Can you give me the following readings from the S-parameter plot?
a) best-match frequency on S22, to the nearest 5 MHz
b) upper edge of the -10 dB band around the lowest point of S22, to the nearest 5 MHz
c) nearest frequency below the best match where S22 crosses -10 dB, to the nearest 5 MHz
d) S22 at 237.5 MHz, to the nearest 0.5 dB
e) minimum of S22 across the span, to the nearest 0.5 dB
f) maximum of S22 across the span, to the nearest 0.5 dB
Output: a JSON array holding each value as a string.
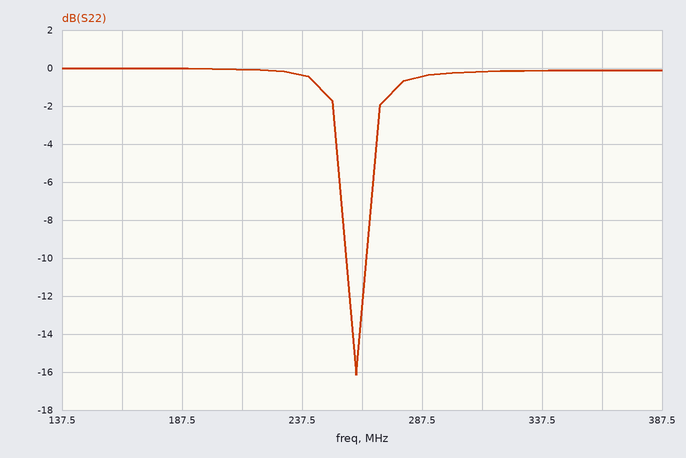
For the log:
["260 MHz", "265 MHz", "255 MHz", "-0.5 dB", "-16.0 dB", "0.0 dB"]
